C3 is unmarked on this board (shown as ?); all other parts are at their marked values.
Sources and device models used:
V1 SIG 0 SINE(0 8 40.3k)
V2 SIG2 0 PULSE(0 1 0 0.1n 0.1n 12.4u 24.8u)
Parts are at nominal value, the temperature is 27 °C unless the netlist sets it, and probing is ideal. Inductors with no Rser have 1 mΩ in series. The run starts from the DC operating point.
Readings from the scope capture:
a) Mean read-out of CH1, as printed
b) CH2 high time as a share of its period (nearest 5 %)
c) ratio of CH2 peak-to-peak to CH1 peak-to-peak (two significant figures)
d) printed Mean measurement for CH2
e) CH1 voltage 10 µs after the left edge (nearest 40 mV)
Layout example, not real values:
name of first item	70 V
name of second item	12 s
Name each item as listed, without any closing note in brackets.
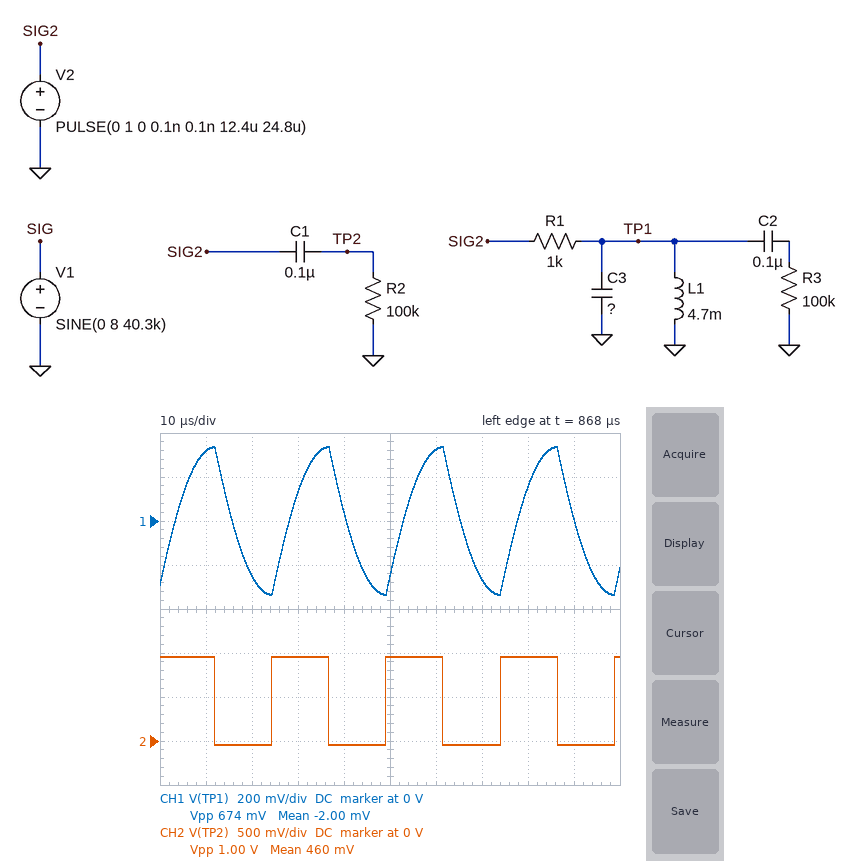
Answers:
Mean read-out of CH1, as printed	-2.00 mV
CH2 high time as a share of its period	50 %
ratio of CH2 peak-to-peak to CH1 peak-to-peak	1.5
printed Mean measurement for CH2	460 mV
CH1 voltage 10 µs after the left edge	320 mV
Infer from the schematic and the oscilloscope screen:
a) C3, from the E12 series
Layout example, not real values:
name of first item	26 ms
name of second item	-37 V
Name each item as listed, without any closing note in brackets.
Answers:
C3, from the E12 series	10 nF
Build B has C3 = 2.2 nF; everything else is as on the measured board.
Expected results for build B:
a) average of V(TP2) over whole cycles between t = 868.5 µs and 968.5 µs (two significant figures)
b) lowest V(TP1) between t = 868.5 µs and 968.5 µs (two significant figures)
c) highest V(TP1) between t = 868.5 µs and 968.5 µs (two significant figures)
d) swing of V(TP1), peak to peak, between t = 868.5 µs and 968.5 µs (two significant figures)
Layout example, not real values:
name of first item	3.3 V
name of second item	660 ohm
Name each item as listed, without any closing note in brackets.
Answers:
average of V(TP2) over whole cycles between t = 868.5 µs and 968.5 µs	460 mV
lowest V(TP1) between t = 868.5 µs and 968.5 µs	-660 mV
highest V(TP1) between t = 868.5 µs and 968.5 µs	660 mV
swing of V(TP1), peak to peak, between t = 868.5 µs and 968.5 µs	1.3 V
